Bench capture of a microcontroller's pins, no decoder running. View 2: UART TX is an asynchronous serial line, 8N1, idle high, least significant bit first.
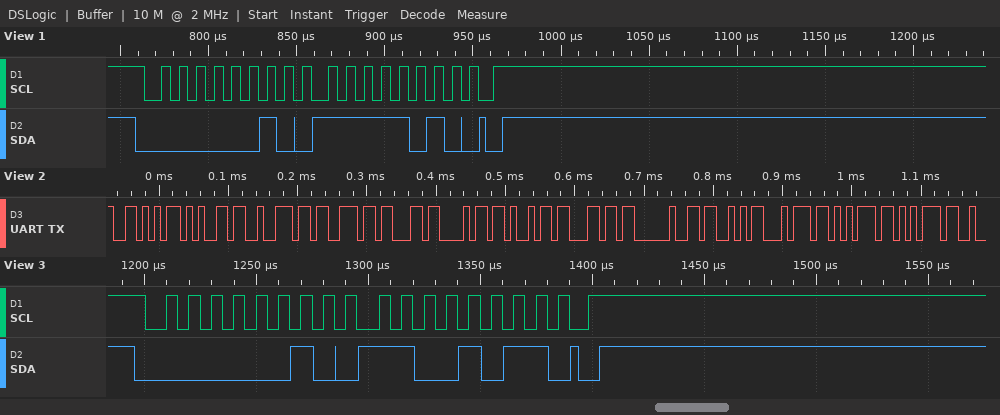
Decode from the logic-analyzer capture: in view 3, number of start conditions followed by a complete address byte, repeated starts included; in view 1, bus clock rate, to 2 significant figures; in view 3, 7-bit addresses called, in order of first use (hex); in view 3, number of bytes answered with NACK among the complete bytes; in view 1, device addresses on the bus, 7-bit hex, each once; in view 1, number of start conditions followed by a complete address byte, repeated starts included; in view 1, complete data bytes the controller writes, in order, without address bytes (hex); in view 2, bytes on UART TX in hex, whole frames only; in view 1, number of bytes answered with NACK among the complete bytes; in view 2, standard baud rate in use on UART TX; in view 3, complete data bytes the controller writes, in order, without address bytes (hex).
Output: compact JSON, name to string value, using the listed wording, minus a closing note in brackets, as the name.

{"in view 3, number of start conditions followed by a complete address byte, repeated starts included": "1", "in view 1, bus clock rate, to 2 significant figures": "100 kHz", "in view 3, 7-bit addresses called, in order of first use": "0x01", "in view 3, number of bytes answered with NACK among the complete bytes": "0", "in view 1, device addresses on the bus, 7-bit hex, each once": "0x01", "in view 1, number of start conditions followed by a complete address byte, repeated starts included": "1", "in view 1, complete data bytes the controller writes, in order, without address bytes": "FA", "in view 2, bytes on UART TX in hex, whole frames only": "56 65 72 73 63 68 69 6C 20 53 74 75 75", "in view 1, number of bytes answered with NACK among the complete bytes": "0", "in view 2, standard baud rate in use on UART TX": "115200 baud", "in view 3, complete data bytes the controller writes, in order, without address bytes": "CB"}
